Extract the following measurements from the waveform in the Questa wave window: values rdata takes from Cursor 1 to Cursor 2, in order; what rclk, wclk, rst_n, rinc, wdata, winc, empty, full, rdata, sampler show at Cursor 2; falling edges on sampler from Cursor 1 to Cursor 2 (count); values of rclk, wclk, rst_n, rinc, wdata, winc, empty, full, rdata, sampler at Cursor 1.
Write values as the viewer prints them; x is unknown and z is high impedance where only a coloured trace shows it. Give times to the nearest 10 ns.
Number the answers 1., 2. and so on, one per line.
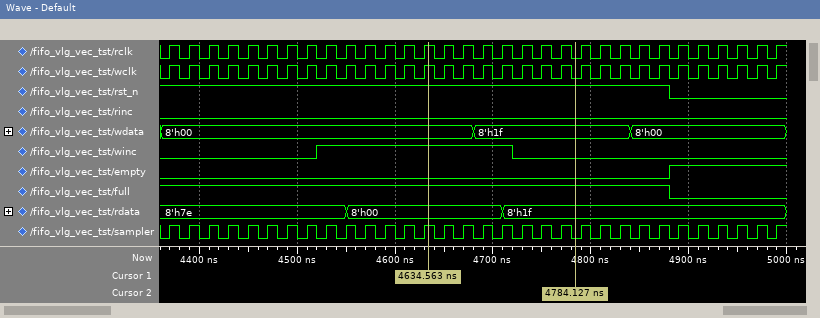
1. 8'h00, 8'h1f
2. rclk=0, wclk=0, rst_n=1, rinc=0, wdata=8'h1f, winc=0, empty=0, full=1, rdata=8'h1f, sampler=0
3. 8
4. rclk=1, wclk=1, rst_n=1, rinc=0, wdata=8'h00, winc=1, empty=0, full=1, rdata=8'h00, sampler=1
